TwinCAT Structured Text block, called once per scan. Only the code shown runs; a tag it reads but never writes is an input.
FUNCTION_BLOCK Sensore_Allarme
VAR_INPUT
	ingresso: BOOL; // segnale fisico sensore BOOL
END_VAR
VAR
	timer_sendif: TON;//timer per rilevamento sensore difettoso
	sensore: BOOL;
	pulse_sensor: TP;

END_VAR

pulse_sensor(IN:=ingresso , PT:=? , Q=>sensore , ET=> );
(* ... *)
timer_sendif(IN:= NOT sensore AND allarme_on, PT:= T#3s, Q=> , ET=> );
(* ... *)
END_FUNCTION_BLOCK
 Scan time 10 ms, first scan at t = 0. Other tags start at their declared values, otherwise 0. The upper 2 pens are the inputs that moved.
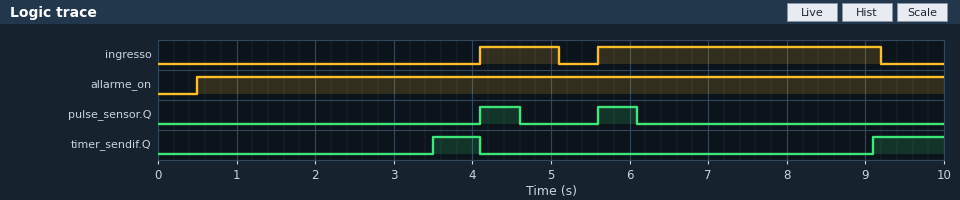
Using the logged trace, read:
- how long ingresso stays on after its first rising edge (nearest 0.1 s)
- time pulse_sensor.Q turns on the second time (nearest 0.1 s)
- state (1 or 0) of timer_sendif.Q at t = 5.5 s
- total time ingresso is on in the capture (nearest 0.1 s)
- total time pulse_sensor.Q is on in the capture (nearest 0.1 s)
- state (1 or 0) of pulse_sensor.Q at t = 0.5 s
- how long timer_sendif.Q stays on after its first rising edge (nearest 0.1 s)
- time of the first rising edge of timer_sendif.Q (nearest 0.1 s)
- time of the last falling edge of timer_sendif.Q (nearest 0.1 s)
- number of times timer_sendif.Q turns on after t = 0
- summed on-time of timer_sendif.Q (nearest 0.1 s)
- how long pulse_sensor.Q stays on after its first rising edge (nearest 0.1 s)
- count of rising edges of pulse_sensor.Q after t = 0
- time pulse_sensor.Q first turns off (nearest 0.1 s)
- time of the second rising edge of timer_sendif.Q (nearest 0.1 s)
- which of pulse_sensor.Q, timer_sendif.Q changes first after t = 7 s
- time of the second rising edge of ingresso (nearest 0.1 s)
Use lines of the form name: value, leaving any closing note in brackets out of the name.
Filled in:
how long ingresso stays on after its first rising edge: 1.0 s
time pulse_sensor.Q turns on the second time: 5.6 s
state (1 or 0) of timer_sendif.Q at t = 5.5 s: 0
total time ingresso is on in the capture: 4.6 s
total time pulse_sensor.Q is on in the capture: 1.0 s
state (1 or 0) of pulse_sensor.Q at t = 0.5 s: 0
how long timer_sendif.Q stays on after its first rising edge: 0.6 s
time of the first rising edge of timer_sendif.Q: 3.5 s
time of the last falling edge of timer_sendif.Q: 4.1 s
number of times timer_sendif.Q turns on after t = 0: 2
summed on-time of timer_sendif.Q: 1.5 s
how long pulse_sensor.Q stays on after its first rising edge: 0.5 s
count of rising edges of pulse_sensor.Q after t = 0: 2
time pulse_sensor.Q first turns off: 4.6 s
time of the second rising edge of timer_sendif.Q: 9.1 s
which of pulse_sensor.Q, timer_sendif.Q changes first after t = 7 s: timer_sendif.Q
time of the second rising edge of ingresso: 5.6 s
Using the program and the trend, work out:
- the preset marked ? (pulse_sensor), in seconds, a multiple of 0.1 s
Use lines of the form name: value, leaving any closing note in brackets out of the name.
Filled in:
the preset marked ? (pulse_sensor), in seconds, a multiple of 0.1 s: 0.5 s
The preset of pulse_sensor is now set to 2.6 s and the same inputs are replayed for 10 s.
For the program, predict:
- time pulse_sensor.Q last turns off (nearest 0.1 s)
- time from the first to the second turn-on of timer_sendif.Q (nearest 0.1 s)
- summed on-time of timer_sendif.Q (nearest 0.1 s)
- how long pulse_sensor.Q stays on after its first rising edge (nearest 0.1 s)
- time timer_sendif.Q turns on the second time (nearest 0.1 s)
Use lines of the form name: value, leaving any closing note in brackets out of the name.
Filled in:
time pulse_sensor.Q last turns off: 6.7 s
time from the first to the second turn-on of timer_sendif.Q: 6.2 s
summed on-time of timer_sendif.Q: 0.9 s
how long pulse_sensor.Q stays on after its first rising edge: 2.6 s
time timer_sendif.Q turns on the second time: 9.7 s
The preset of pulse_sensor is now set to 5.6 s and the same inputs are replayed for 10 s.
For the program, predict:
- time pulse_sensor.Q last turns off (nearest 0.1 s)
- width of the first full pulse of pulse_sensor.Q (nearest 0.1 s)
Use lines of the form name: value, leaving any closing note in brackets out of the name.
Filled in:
time pulse_sensor.Q last turns off: 9.7 s
width of the first full pulse of pulse_sensor.Q: 5.6 s
